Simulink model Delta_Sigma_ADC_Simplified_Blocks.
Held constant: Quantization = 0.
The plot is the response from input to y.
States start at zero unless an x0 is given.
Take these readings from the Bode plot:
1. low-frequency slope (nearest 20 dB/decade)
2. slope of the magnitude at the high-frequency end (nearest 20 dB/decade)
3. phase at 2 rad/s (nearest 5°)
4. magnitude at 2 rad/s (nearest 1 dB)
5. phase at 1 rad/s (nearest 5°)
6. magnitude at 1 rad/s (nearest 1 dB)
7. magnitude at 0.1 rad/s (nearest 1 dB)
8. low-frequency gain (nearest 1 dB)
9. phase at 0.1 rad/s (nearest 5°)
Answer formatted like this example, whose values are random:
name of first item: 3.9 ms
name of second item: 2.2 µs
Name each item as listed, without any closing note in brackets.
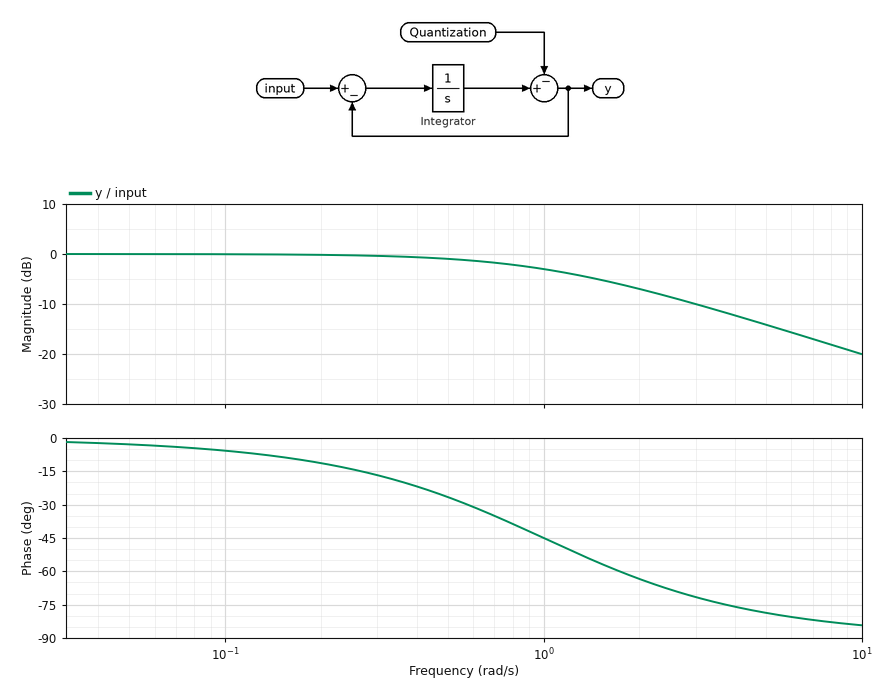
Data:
low-frequency slope: 0 dB/decade
slope of the magnitude at the high-frequency end: -20 dB/decade
phase at 2 rad/s: -65°
magnitude at 2 rad/s: -7 dB
phase at 1 rad/s: -45°
magnitude at 1 rad/s: -3 dB
magnitude at 0.1 rad/s: 0 dB
low-frequency gain: 0 dB
phase at 0.1 rad/s: -5°
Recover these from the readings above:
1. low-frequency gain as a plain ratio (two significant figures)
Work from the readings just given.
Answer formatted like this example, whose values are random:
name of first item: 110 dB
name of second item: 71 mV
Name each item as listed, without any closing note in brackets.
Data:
low-frequency gain as a plain ratio: 1.0
